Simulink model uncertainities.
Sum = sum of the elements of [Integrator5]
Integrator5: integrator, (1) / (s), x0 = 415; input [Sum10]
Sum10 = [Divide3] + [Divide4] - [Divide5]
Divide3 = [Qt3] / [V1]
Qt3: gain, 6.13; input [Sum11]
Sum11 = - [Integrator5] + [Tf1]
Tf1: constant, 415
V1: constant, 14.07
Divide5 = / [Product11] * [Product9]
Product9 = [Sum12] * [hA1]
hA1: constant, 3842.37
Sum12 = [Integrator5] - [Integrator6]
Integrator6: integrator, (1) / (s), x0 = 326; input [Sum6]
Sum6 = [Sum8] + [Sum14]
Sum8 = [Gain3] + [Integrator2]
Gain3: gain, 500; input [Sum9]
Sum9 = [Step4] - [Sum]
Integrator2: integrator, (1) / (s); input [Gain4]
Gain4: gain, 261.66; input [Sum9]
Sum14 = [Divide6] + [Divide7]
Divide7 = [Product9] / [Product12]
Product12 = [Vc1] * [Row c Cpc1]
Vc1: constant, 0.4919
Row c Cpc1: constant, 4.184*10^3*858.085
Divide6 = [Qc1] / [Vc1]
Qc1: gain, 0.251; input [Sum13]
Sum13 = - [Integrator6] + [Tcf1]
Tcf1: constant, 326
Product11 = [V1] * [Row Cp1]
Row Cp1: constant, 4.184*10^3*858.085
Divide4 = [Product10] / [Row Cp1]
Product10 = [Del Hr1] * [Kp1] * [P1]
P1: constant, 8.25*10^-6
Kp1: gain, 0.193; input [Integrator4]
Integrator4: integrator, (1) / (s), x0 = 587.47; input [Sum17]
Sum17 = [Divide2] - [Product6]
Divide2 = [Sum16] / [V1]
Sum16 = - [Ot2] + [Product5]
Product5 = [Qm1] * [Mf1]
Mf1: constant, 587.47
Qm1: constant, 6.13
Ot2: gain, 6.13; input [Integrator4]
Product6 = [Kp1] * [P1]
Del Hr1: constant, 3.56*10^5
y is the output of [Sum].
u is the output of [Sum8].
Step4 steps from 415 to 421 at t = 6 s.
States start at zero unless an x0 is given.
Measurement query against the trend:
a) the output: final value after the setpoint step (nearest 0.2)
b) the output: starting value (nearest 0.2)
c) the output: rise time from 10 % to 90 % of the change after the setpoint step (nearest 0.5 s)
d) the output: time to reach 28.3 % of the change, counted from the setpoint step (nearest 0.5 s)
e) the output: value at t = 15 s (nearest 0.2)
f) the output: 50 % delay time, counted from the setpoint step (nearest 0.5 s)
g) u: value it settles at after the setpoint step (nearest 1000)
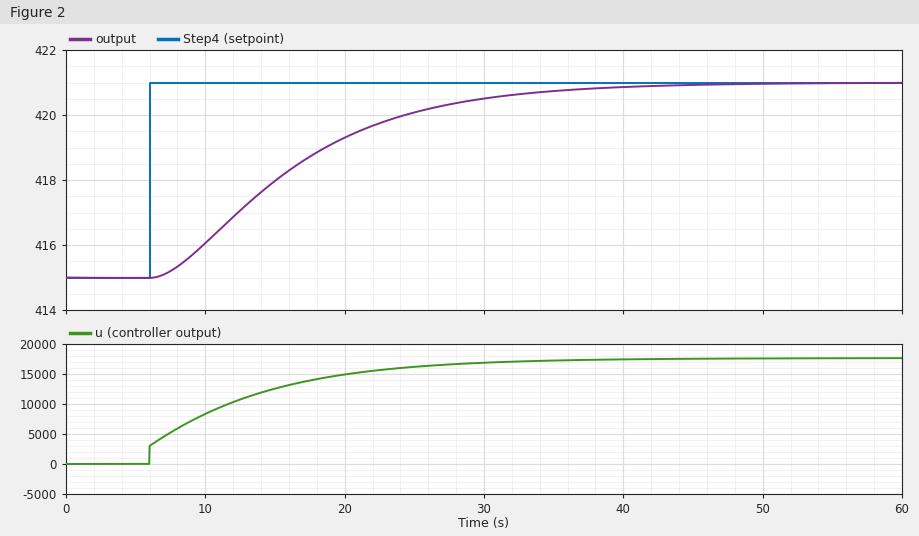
421.0
415.0
19.5 s
5.5 s
418.0
9.0 s
18000
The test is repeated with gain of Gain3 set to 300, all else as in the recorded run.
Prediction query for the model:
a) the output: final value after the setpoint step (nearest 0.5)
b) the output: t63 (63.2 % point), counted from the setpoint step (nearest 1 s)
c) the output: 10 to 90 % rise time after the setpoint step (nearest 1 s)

421.0
12 s
18 s
